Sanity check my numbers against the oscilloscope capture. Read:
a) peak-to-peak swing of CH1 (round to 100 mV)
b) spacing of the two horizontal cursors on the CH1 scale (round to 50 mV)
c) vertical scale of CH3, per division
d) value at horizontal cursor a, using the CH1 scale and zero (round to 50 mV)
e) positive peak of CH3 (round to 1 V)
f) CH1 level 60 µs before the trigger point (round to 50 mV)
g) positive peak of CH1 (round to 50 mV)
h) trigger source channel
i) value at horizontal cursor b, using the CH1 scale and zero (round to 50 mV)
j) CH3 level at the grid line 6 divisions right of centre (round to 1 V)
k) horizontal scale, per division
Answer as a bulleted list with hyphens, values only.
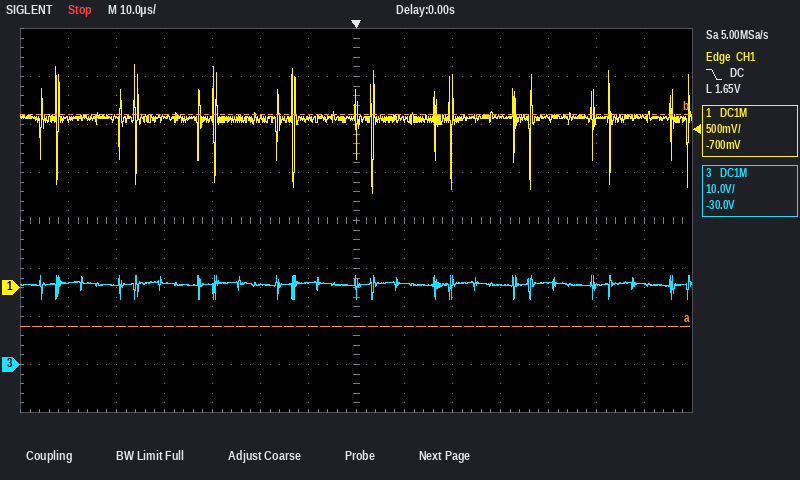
- 1.30 V
- 2.20 V
- 10 V
- -400 mV
- 19 V
- 1.75 V
- 2.30 V
- CH1
- 1.80 V
- 17 V
- 10 µs
